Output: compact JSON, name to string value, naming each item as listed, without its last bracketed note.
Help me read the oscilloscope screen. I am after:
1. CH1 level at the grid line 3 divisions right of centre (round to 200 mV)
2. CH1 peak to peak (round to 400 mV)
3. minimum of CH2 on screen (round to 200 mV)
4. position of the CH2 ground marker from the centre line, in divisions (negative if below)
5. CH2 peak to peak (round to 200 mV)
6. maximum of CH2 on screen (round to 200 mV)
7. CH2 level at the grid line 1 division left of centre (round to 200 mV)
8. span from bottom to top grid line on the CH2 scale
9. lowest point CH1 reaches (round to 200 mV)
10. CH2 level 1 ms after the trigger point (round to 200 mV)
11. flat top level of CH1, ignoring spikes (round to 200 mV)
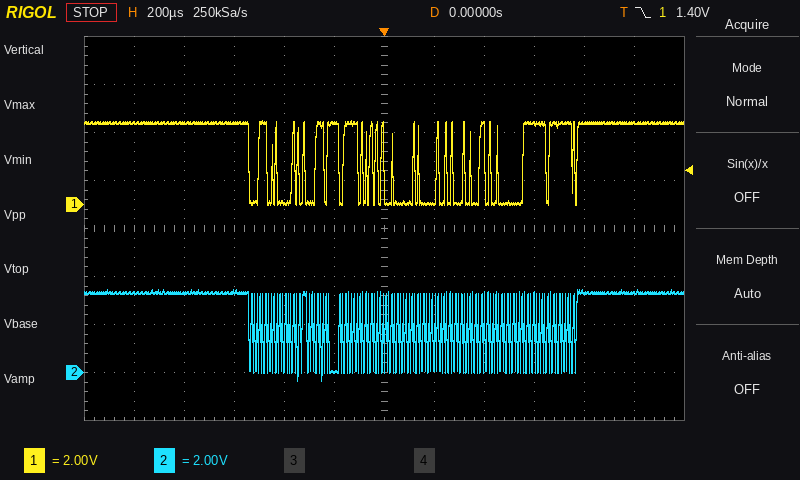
{"CH1 level at the grid line 3 divisions right of centre": "3.4 V", "CH1 peak to peak": "3.6 V", "minimum of CH2 on screen": "-400 mV", "position of the CH2 ground marker from the centre line, in divisions": "-3.0 div", "CH2 peak to peak": "3.8 V", "maximum of CH2 on screen": "3.4 V", "CH2 level at the grid line 1 division left of centre": "0.0 V", "span from bottom to top grid line on the CH2 scale": "16 V", "lowest point CH1 reaches": "0.0 V", "CH2 level 1 ms after the trigger point": "3.4 V", "flat top level of CH1, ignoring spikes": "3.4 V"}
